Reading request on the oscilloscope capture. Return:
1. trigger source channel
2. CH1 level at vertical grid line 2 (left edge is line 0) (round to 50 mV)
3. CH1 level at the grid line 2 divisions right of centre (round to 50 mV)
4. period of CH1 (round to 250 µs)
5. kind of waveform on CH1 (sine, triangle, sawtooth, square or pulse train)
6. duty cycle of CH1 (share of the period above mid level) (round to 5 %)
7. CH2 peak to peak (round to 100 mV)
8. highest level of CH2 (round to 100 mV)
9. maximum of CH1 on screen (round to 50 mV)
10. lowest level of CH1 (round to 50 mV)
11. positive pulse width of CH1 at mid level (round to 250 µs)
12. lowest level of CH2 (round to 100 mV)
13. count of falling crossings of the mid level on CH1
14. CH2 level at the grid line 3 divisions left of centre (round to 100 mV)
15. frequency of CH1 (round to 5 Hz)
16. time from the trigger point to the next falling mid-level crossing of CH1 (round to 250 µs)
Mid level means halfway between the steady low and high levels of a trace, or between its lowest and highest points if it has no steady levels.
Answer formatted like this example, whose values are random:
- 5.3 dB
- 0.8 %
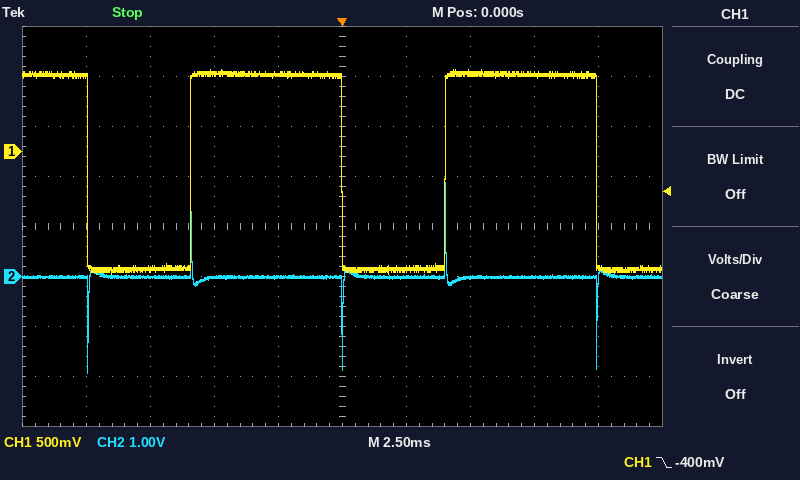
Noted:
- CH1
- -1.15 V
- 800 mV
- 10.00 ms
- pulse train
- 60 %
- 3.8 V
- 1.9 V
- 800 mV
- -1.20 V
- 6.00 ms
- -1.9 V
- 3
- 0.0 V
- 100 Hz
- 10.00 ms
